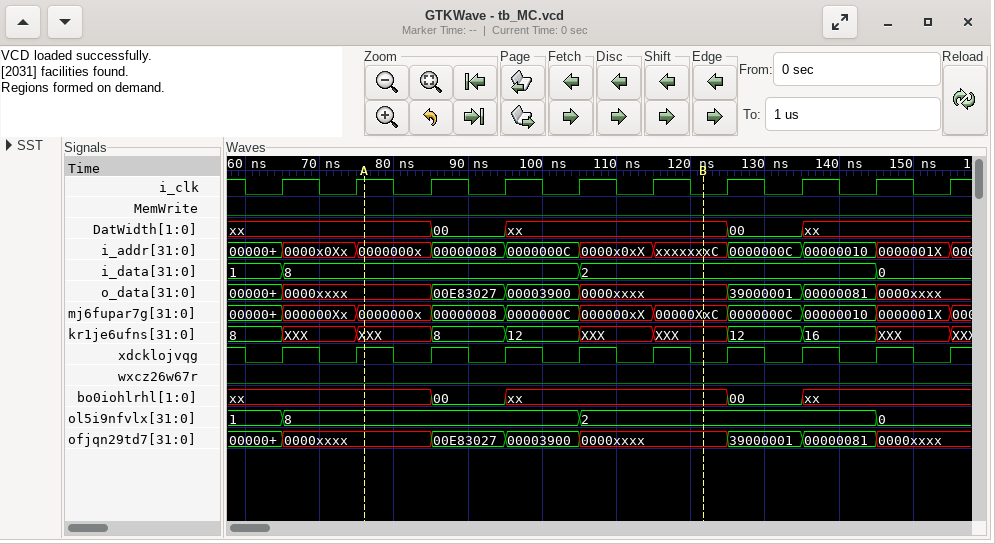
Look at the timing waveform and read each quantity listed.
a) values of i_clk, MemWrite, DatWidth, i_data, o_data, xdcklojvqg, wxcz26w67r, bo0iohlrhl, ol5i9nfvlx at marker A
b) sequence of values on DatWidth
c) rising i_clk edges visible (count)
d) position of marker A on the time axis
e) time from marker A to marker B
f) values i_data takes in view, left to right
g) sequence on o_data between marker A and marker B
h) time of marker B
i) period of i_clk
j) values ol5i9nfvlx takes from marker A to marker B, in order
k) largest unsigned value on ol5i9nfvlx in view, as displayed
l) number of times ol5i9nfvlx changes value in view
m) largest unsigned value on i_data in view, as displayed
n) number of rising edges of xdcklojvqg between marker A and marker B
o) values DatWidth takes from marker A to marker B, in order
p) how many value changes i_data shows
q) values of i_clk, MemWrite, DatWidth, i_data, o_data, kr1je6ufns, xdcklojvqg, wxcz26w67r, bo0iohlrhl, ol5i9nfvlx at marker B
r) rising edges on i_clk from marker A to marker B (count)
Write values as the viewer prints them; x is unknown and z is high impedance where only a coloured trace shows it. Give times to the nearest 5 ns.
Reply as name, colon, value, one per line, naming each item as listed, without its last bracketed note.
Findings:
values of i_clk, MemWrite, DatWidth, i_data, o_data, xdcklojvqg, wxcz26w67r, bo0iohlrhl, ol5i9nfvlx at marker A: i_clk=1, MemWrite=0, DatWidth=xx, i_data=8, o_data=0000xxxx, xdcklojvqg=1, wxcz26w67r=0, bo0iohlrhl=xx, ol5i9nfvlx=8
sequence of values on DatWidth: xx, 00, xx, 00, xx
rising i_clk edges visible: 10
position of marker A on the time axis: 75 ns
time from marker A to marker B: 45 ns
values i_data takes in view, left to right: 1, 8, 2, 0
sequence on o_data between marker A and marker B: 0000xxxx, 00E83027, 00003900, 0000xxxx
time of marker B: 120 ns
period of i_clk: 10 ns
values ol5i9nfvlx takes from marker A to marker B, in order: 8, 2
largest unsigned value on ol5i9nfvlx in view, as displayed: 8
number of times ol5i9nfvlx changes value in view: 3
largest unsigned value on i_data in view, as displayed: 8
number of rising edges of xdcklojvqg between marker A and marker B: 4
values DatWidth takes from marker A to marker B, in order: xx, 00, xx
how many value changes i_data shows: 3
values of i_clk, MemWrite, DatWidth, i_data, o_data, kr1je6ufns, xdcklojvqg, wxcz26w67r, bo0iohlrhl, ol5i9nfvlx at marker B: i_clk=0, MemWrite=0, DatWidth=xx, i_data=2, o_data=0000xxxx, kr1je6ufns=XXX, xdcklojvqg=0, wxcz26w67r=0, bo0iohlrhl=xx, ol5i9nfvlx=2
rising edges on i_clk from marker A to marker B: 4
